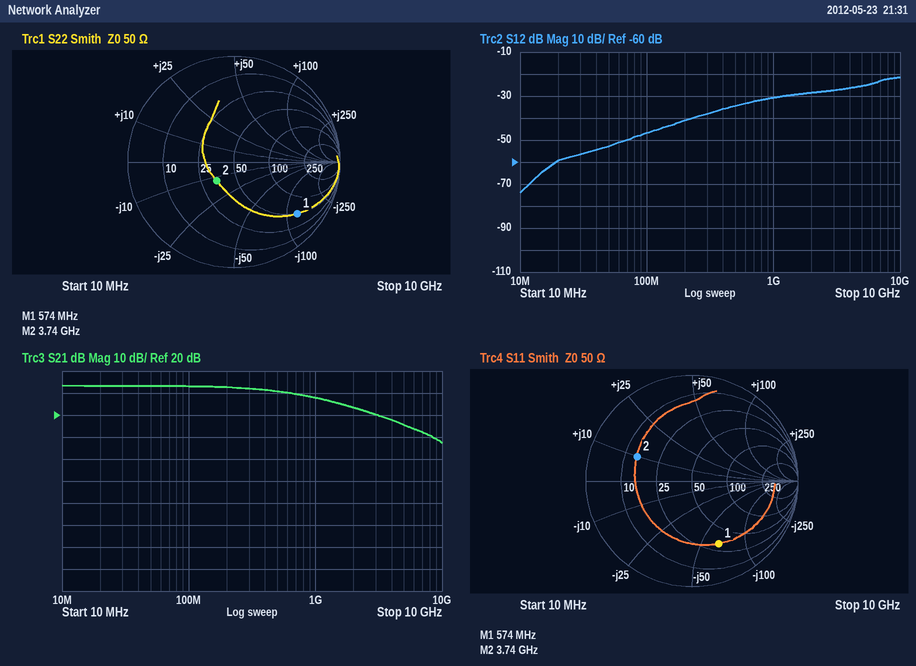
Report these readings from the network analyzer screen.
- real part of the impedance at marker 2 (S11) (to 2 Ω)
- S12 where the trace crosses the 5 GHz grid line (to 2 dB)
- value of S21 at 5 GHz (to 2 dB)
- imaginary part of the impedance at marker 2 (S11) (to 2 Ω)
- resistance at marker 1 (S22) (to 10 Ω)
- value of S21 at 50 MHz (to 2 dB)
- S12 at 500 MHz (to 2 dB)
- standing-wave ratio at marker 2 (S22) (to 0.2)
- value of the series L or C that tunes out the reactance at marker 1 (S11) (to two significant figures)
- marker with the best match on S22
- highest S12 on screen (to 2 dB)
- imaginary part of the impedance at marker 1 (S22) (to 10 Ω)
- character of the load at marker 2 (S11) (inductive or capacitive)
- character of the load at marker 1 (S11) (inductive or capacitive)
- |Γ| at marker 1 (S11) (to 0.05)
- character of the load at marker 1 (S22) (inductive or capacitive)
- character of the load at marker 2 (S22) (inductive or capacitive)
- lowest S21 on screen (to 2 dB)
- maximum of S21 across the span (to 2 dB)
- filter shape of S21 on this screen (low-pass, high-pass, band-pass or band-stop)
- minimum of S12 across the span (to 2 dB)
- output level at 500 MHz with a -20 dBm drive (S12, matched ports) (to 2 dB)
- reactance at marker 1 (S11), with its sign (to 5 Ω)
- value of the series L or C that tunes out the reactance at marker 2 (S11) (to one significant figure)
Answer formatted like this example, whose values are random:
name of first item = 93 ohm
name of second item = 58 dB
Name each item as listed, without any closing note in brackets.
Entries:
real part of the impedance at marker 2 (S11) = 14 Ω
S12 where the trace crosses the 5 GHz grid line = -26 dB
value of S21 at 5 GHz = 16 dB
imaginary part of the impedance at marker 2 (S11) = +10 Ω
resistance at marker 1 (S22) = 50 Ω
value of S21 at 50 MHz = 34 dB
S12 at 500 MHz = -34 dB
standing-wave ratio at marker 2 (S22) = 1.6
value of the series L or C that tunes out the reactance at marker 1 (S11) = 18 nH
marker with the best match on S22 = marker 2
highest S12 on screen = -22 dB
imaginary part of the impedance at marker 1 (S22) = -120 Ω
character of the load at marker 2 (S11) = inductive
character of the load at marker 1 (S11) = capacitive
|Γ| at marker 1 (S11) = 0.65
character of the load at marker 1 (S22) = capacitive
character of the load at marker 2 (S22) = capacitive
lowest S21 on screen = 8 dB
maximum of S21 across the span = 34 dB
filter shape of S21 on this screen = low-pass
minimum of S12 across the span = -74 dB
output level at 500 MHz with a -20 dBm drive (S12, matched ports) = -54 dBm
reactance at marker 1 (S11), with its sign = -65 Ω
value of the series L or C that tunes out the reactance at marker 2 (S11) = 4 pF
